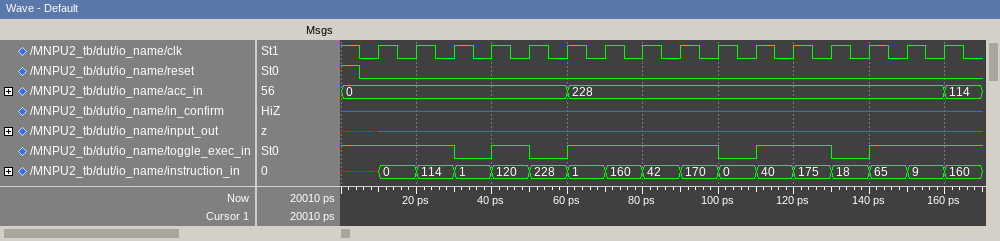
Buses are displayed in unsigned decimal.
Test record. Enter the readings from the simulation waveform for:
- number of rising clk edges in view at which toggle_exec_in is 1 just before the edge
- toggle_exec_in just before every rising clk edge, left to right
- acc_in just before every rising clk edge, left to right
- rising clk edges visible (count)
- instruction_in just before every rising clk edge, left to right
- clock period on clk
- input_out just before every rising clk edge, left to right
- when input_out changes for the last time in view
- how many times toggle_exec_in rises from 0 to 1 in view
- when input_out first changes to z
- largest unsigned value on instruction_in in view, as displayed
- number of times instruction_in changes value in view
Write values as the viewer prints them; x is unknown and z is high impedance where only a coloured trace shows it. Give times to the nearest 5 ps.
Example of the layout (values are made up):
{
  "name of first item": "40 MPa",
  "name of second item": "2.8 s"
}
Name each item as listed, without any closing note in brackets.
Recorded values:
{
  "number of rising clk edges in view at which toggle_exec_in is 1 just before the edge": "12",
  "toggle_exec_in just before every rising clk edge, left to right": "1 1 1 0 1 0 1 1 1 1 0 1 1 0 1 1",
  "acc_in just before every rising clk edge, left to right": "0, 0, 0, 0, 0, 0, 228, 228, 228, 228, 228, 228, 228, 228, 228, 228",
  "rising clk edges visible": "16",
  "instruction_in just before every rising clk edge, left to right": "x, 0, 114, 1, 120, 228, 1, 160, 42, 170, 0, 40, 175, 18, 65, 9",
  "clock period on clk": "10 ps",
  "input_out just before every rising clk edge, left to right": "x, z, z, z, z, z, z, z, z, z, z, z, z, z, z, z",
  "when input_out changes for the last time in view": "10 ps",
  "how many times toggle_exec_in rises from 0 to 1 in view": "4",
  "when input_out first changes to z": "10 ps",
  "largest unsigned value on instruction_in in view, as displayed": "228",
  "number of times instruction_in changes value in view": "16"
}
